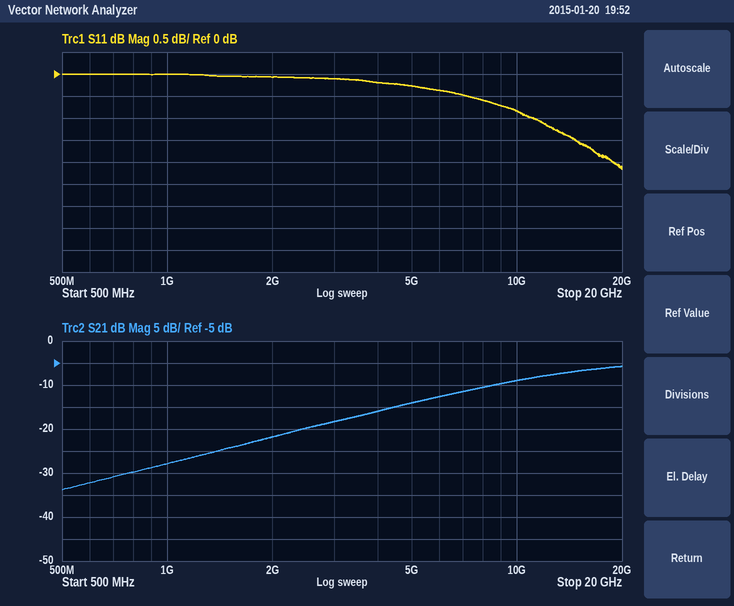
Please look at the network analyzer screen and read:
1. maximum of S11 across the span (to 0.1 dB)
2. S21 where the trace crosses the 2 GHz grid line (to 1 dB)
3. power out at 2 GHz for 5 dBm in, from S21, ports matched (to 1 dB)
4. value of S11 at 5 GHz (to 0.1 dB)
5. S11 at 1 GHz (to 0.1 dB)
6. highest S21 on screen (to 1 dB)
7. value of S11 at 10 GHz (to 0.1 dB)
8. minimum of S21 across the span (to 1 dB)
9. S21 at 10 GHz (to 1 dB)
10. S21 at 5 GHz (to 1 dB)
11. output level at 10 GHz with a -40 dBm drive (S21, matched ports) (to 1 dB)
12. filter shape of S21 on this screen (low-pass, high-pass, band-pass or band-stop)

0.0 dB
-22 dB
-17 dBm
-0.3 dB
0.0 dB
-6 dB
-0.8 dB
-34 dB
-9 dB
-14 dB
-49 dBm
high-pass
